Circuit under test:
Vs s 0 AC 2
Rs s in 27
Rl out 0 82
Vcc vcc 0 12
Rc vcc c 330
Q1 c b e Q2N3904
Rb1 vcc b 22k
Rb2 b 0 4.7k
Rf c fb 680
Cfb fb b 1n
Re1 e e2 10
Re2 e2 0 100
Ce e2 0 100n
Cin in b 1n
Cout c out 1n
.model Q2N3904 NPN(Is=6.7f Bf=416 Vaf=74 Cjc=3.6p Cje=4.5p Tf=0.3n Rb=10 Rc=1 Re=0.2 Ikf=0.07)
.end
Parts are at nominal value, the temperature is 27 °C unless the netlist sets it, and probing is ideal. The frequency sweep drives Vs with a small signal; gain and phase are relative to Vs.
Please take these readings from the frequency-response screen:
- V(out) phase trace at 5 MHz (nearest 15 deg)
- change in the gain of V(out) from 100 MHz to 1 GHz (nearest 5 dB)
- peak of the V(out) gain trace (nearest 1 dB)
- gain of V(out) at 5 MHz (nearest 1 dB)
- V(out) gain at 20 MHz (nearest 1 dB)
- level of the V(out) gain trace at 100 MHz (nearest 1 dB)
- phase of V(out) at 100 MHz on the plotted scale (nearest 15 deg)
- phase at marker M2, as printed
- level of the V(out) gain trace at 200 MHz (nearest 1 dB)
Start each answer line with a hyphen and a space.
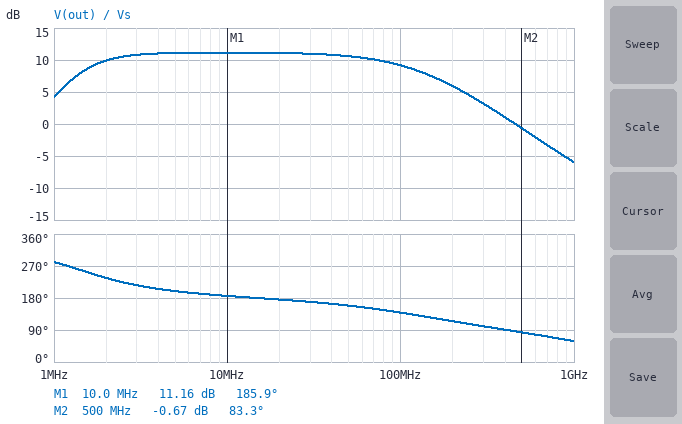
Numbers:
- 195 deg
- -15 dB
- 11 dB
- 11 dB
- 11 dB
- 9 dB
- 135 deg
- 83.3 deg
- 6 dB
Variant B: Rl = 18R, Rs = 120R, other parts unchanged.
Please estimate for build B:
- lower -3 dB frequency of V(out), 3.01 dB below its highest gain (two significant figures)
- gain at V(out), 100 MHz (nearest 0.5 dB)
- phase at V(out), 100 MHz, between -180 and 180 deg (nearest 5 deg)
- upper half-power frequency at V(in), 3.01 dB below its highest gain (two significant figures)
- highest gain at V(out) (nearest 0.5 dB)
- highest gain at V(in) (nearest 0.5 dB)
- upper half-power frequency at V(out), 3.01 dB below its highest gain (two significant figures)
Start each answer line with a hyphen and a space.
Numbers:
- 1.8 MHz
- -7.5 dB
- 120 deg
- 870 kHz
- -1.5 dB
- 0 dB
- 60 MHz
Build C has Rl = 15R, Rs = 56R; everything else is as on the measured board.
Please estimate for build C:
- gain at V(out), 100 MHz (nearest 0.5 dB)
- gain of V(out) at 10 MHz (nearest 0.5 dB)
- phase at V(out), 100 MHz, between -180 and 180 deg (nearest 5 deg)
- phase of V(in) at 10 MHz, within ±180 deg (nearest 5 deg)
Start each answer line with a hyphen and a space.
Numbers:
- -4.5 dB
- -1.0 dB
- 130 deg
- 0 deg
